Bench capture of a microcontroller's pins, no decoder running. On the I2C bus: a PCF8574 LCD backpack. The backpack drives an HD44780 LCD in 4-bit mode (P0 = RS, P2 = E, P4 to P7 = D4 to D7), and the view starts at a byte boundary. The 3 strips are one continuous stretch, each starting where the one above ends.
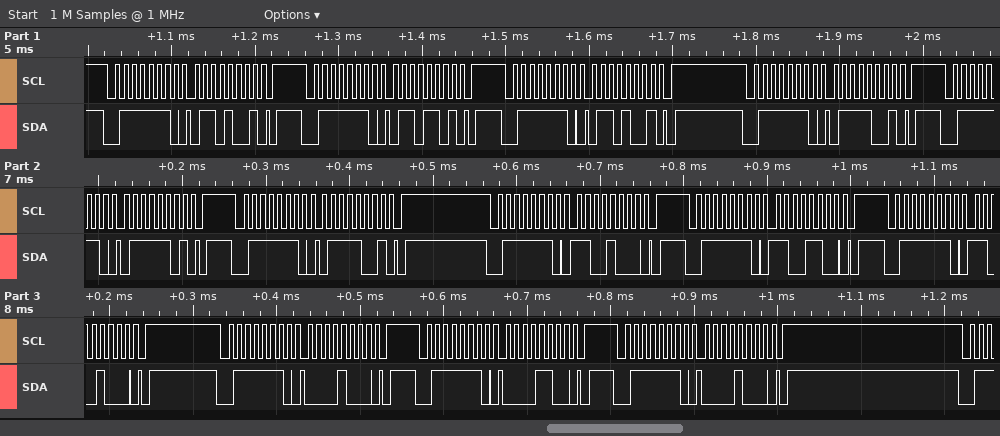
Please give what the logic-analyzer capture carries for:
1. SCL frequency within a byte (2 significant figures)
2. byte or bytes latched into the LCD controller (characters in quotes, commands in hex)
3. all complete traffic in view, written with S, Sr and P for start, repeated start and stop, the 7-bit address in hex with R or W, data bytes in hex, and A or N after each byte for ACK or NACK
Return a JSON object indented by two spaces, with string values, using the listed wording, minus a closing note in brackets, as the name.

{
  "SCL frequency within a byte": "100 kHz",
  "byte or bytes latched into the LCD controller": "'g' 0xC0",
  "all complete traffic in view, written with S, Sr and P for start, repeated start and stop, the 7-bit address in hex with R or W, data bytes in hex, and A or N after each byte for ACK or NACK": "S 3FW A 69 A P S 3FW A 6D A P S 3FW A 69 A P S 3FW A 79 A P S 3FW A 7D A P S 3FW A 79 A P S 3FW A C8 A P S 3FW A CC A P S 3FW A C8 A P S 3FW A 08 A P S 3FW A 0C A P S 3FW A 08 A P"
}
